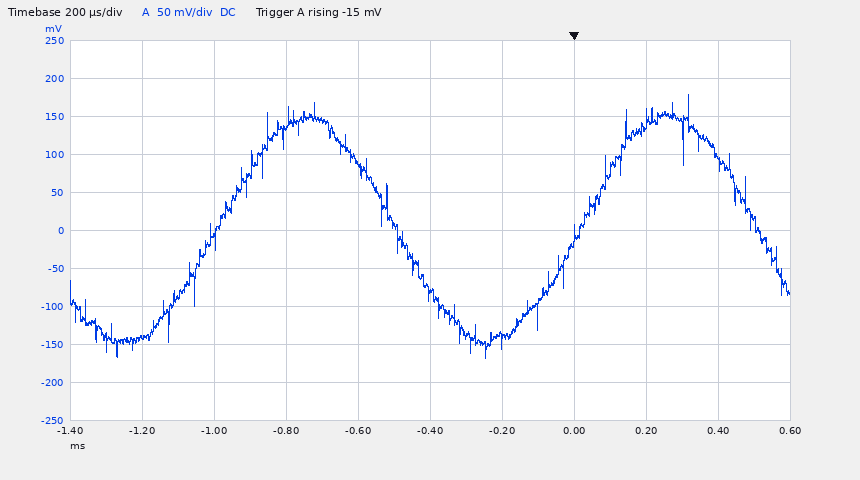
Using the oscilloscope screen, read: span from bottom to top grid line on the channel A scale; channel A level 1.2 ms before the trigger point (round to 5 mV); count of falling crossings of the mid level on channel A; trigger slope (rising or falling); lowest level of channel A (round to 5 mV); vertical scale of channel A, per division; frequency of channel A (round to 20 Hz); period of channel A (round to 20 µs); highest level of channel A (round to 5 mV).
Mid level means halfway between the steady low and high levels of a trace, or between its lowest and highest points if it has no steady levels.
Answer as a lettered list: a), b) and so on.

a) 500 mV
b) -140 mV
c) 2
d) rising
e) -170 mV
f) 50 mV
g) 1.00 kHz
h) 1.00 ms
i) 180 mV
